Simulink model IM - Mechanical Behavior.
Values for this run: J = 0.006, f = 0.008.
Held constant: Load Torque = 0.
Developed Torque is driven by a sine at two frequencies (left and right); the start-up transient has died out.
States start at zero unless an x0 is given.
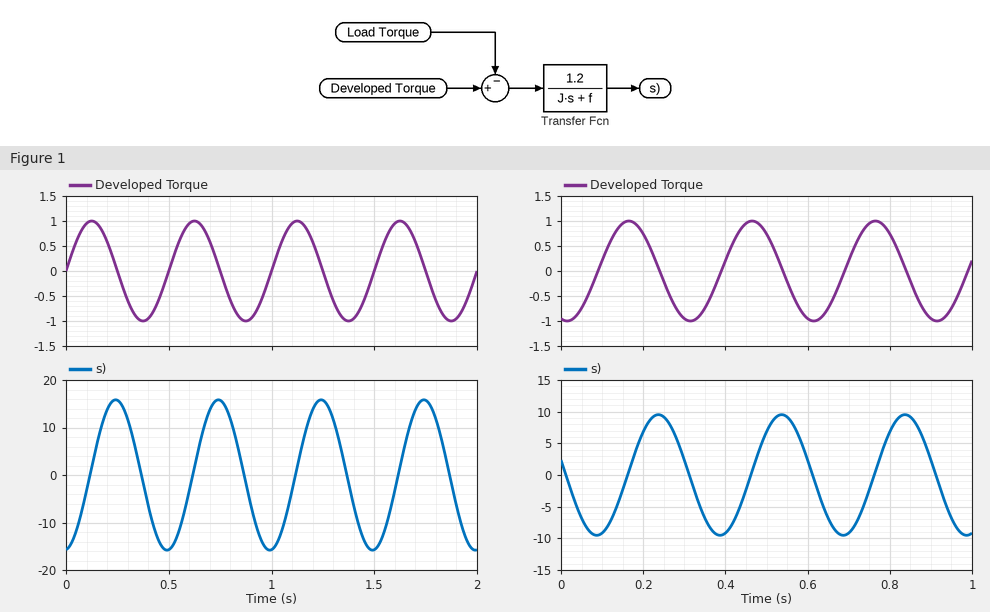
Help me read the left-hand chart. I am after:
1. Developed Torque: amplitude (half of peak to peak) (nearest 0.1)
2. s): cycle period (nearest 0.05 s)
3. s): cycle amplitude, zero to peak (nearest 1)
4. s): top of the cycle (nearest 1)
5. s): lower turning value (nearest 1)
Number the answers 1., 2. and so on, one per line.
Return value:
1. 1.0
2. 0.50 s
3. 16
4. 16
5. -16
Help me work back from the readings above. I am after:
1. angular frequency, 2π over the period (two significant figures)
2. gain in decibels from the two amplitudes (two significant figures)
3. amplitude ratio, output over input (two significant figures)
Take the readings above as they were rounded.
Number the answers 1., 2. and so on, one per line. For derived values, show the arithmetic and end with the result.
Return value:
1. 2π / 0.5 = 13 rad/s
2. 20 log10(16 / 1) = 24 dB
3. 16 / 1 = 16
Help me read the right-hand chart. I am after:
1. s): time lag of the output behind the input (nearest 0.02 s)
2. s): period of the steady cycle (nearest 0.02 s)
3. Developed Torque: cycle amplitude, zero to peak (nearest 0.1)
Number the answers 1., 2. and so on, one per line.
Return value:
1. 0.08 s
2. 0.30 s
3. 1.0
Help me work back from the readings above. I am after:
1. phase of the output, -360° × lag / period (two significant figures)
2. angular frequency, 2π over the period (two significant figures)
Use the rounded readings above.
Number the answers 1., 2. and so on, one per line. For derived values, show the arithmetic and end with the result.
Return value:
1. -360 × 0.08 / 0.3 = -96°
2. 2π / 0.3 = 21 rad/s
